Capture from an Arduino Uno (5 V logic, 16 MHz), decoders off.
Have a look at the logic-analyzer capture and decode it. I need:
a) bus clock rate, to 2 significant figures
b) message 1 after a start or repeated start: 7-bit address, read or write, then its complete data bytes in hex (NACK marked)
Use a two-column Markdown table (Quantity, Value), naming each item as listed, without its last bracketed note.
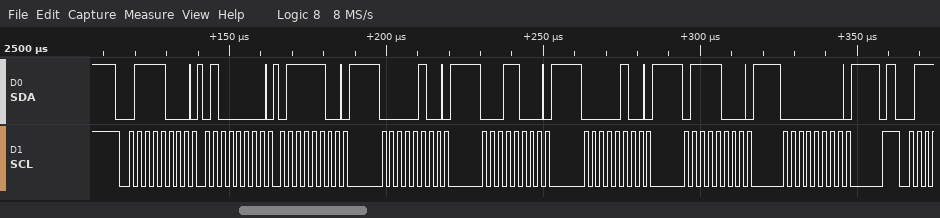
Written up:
| Quantity | Value |
|---|---|
| bus clock rate, to 2 significant figures | 400 kHz |
| message 1 after a start or repeated start: 7-bit address, read or write, then its complete data bytes in hex | 0x3C write: 40 7C 04 18 04 78 00 |
